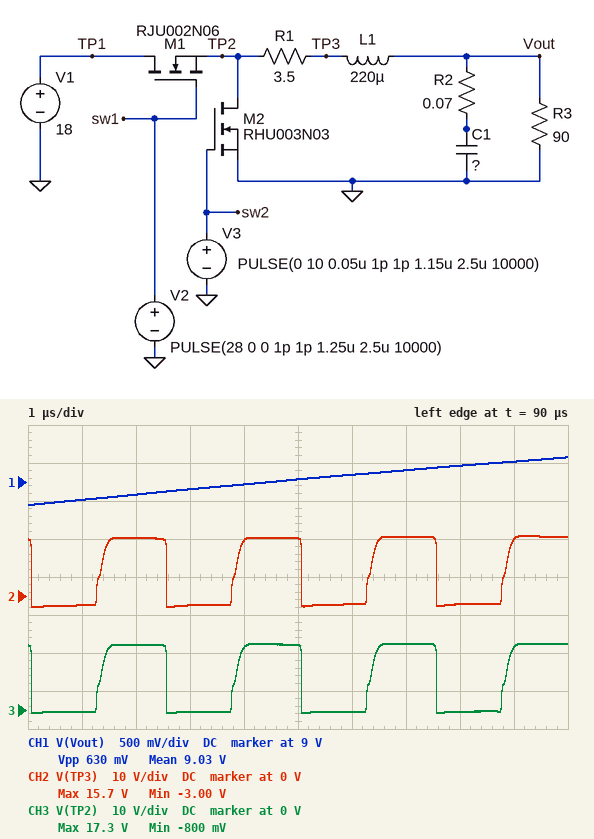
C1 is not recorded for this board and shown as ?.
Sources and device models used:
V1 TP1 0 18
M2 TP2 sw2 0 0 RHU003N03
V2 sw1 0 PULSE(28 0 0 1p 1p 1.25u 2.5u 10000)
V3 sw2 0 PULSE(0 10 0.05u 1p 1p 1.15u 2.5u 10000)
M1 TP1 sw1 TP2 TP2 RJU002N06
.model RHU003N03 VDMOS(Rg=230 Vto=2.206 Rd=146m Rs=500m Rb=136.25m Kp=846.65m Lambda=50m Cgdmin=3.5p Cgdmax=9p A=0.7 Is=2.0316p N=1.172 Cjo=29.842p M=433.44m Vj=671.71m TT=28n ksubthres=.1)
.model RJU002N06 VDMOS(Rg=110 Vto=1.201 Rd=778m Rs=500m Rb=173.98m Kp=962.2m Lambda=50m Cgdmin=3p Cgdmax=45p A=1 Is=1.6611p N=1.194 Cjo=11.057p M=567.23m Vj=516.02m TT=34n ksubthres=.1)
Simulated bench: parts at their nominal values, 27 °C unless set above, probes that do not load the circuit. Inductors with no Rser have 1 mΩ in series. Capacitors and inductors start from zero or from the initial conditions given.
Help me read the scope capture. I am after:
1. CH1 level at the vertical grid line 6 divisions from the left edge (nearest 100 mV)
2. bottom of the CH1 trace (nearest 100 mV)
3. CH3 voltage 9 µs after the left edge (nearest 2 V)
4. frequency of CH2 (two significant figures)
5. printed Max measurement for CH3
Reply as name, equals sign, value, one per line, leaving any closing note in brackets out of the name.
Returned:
CH1 level at the vertical grid line 6 divisions from the left edge = 9.1 V
bottom of the CH1 trace = 8.7 V
CH3 voltage 9 µs after the left edge = 16 V
frequency of CH2 = 400 kHz
printed Max measurement for CH3 = 17.3 V
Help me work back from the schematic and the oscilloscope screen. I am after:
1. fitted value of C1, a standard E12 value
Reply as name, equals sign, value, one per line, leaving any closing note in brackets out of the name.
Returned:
fitted value of C1, a standard E12 value = 6.8 µF
